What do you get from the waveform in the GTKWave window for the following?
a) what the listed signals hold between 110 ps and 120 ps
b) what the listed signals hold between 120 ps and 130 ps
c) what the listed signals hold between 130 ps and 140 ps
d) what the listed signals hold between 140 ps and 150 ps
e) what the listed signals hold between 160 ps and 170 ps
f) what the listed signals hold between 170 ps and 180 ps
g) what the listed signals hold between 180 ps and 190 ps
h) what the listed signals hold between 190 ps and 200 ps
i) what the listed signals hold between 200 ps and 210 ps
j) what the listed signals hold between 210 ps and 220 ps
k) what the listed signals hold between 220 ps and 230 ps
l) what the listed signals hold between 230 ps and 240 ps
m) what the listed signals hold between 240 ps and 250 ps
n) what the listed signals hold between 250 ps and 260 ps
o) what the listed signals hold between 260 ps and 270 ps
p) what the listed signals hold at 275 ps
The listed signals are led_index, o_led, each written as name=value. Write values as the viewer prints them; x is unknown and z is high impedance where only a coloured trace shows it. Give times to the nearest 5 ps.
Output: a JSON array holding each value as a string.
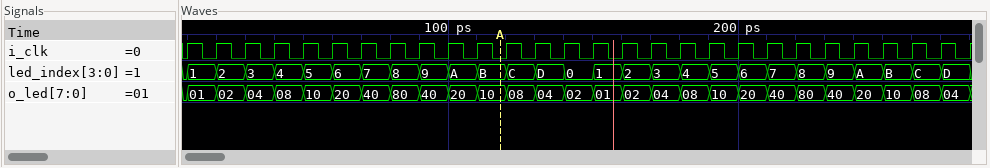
["led_index=B, o_led=10", "led_index=C, o_led=08", "led_index=D, o_led=04", "led_index=0, o_led=02", "led_index=2, o_led=02", "led_index=3, o_led=04", "led_index=4, o_led=08", "led_index=5, o_led=10", "led_index=6, o_led=20", "led_index=7, o_led=40", "led_index=8, o_led=80", "led_index=9, o_led=40", "led_index=A, o_led=20", "led_index=B, o_led=10", "led_index=C, o_led=08", "led_index=D, o_led=04"]
